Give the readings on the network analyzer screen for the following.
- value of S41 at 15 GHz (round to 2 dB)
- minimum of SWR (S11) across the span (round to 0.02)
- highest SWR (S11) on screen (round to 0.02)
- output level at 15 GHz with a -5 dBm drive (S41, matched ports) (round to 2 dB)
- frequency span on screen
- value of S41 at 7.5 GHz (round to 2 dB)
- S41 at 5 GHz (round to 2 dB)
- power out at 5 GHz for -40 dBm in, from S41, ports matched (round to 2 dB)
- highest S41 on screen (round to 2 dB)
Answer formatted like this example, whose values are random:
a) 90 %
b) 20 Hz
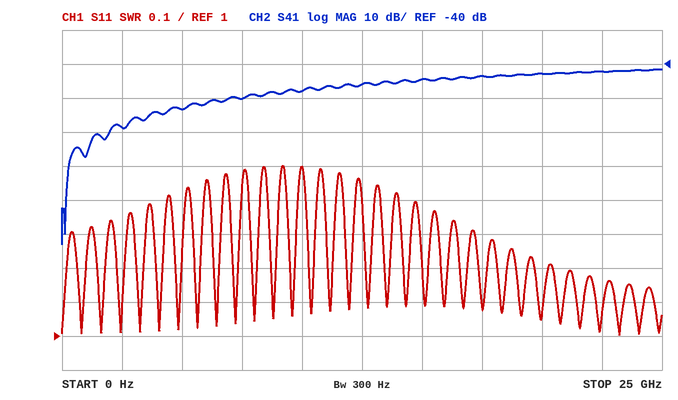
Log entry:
a) -44 dB
b) 1.00
c) 1.50
d) -50 dBm
e) 25 GHz
f) -50 dB
g) -54 dB
h) -94 dBm
i) -42 dB
